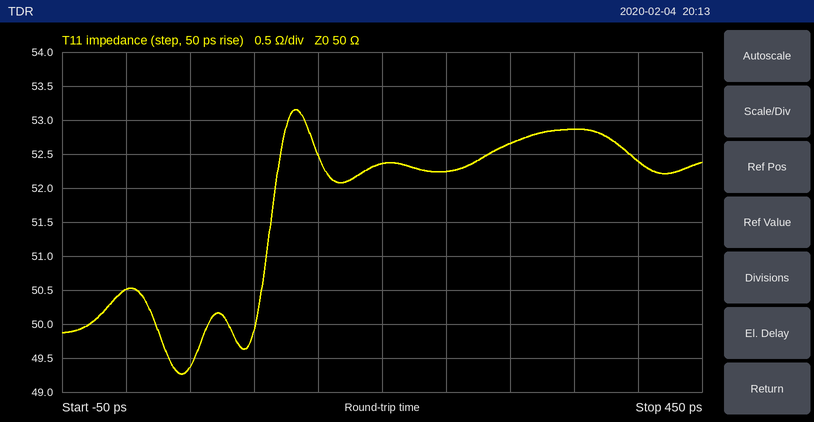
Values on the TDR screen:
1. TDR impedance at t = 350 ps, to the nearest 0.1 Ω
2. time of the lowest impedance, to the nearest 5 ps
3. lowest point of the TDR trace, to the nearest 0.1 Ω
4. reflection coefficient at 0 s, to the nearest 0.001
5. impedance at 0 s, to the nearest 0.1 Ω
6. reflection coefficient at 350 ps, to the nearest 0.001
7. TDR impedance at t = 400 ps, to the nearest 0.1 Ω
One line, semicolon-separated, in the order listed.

52.9 Ω; 45 ps; 49.3 Ω; +0.005; 50.5 Ω; +0.028; 52.4 Ω
